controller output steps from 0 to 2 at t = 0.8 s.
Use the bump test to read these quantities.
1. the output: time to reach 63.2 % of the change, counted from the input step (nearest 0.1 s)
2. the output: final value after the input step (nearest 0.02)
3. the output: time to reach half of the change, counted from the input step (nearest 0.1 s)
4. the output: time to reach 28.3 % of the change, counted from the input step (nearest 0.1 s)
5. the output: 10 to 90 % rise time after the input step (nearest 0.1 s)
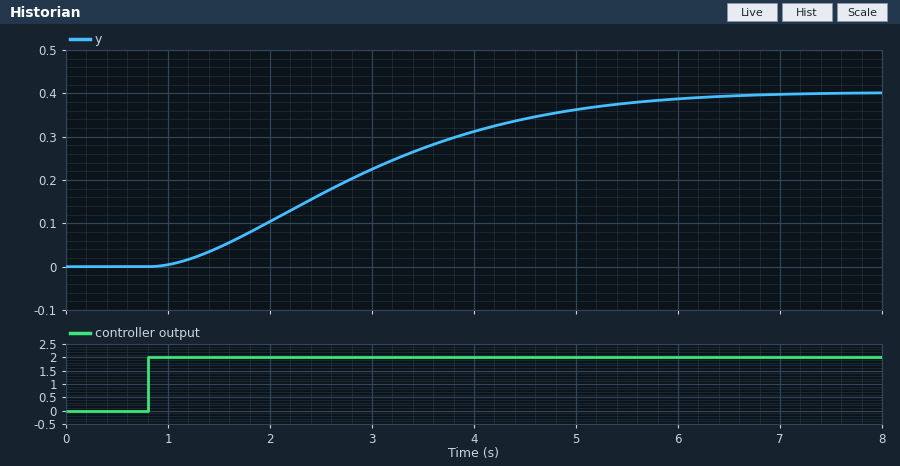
2.5 s
0.40
2.0 s
1.3 s
3.5 s
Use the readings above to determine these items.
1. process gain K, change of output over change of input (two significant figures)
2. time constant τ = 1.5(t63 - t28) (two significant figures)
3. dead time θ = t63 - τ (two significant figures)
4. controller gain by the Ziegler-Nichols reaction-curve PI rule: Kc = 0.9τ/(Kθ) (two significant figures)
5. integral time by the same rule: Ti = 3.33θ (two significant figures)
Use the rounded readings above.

0.20
1.8 s
0.70 s
12
2.3 s
